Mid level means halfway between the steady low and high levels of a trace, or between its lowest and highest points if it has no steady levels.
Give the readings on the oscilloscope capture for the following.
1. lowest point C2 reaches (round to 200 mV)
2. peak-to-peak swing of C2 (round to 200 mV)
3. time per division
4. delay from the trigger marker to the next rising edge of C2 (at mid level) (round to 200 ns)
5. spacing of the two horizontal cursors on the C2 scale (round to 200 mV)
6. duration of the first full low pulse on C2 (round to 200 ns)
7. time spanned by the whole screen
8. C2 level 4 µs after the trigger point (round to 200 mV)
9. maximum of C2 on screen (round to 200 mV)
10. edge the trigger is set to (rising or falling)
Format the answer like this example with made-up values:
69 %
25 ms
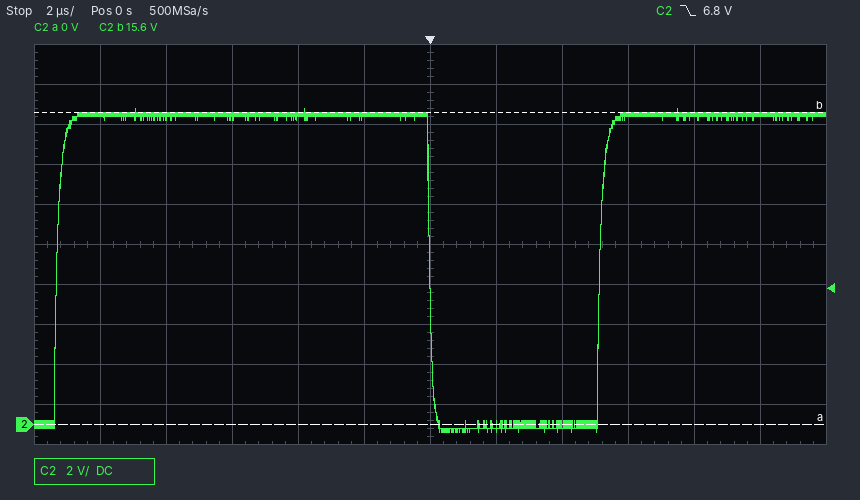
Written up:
-400 mV
16.2 V
2 µs
5.2 µs
15.6 V
5.2 µs
24 µs
0.0 V
15.8 V
falling
